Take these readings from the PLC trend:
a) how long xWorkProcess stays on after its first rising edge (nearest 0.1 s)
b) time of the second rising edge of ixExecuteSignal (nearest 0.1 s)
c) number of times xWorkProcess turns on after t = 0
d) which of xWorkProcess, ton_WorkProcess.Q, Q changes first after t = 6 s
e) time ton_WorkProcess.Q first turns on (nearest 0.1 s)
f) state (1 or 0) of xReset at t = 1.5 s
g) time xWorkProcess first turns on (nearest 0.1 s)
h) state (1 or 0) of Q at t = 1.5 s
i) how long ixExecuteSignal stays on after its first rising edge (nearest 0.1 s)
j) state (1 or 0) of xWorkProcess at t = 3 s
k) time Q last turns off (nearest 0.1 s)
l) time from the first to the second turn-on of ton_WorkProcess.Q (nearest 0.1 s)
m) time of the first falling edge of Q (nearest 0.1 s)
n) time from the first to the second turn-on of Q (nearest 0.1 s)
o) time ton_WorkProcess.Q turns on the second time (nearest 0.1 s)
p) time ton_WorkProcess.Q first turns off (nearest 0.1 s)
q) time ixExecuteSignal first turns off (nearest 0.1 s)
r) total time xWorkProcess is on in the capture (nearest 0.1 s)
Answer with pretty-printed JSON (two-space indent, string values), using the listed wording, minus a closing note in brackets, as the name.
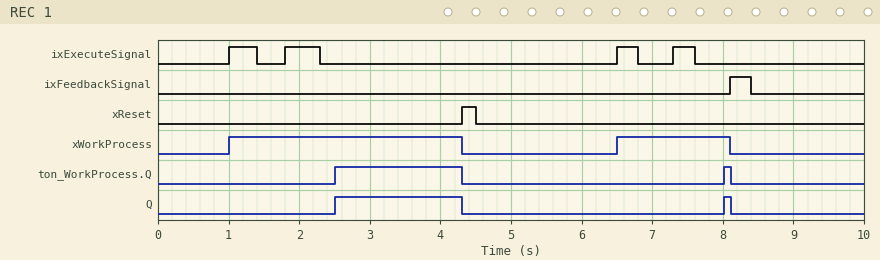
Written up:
{
  "how long xWorkProcess stays on after its first rising edge": "3.3 s",
  "time of the second rising edge of ixExecuteSignal": "1.8 s",
  "number of times xWorkProcess turns on after t = 0": "2",
  "which of xWorkProcess, ton_WorkProcess.Q, Q changes first after t = 6 s": "xWorkProcess",
  "time ton_WorkProcess.Q first turns on": "2.5 s",
  "state (1 or 0) of xReset at t = 1.5 s": "0",
  "time xWorkProcess first turns on": "1.0 s",
  "state (1 or 0) of Q at t = 1.5 s": "0",
  "how long ixExecuteSignal stays on after its first rising edge": "0.4 s",
  "state (1 or 0) of xWorkProcess at t = 3 s": "1",
  "time Q last turns off": "8.1 s",
  "time from the first to the second turn-on of ton_WorkProcess.Q": "5.5 s",
  "time of the first falling edge of Q": "4.3 s",
  "time from the first to the second turn-on of Q": "5.5 s",
  "time ton_WorkProcess.Q turns on the second time": "8.0 s",
  "time ton_WorkProcess.Q first turns off": "4.3 s",
  "time ixExecuteSignal first turns off": "1.4 s",
  "total time xWorkProcess is on in the capture": "4.9 s"
}
